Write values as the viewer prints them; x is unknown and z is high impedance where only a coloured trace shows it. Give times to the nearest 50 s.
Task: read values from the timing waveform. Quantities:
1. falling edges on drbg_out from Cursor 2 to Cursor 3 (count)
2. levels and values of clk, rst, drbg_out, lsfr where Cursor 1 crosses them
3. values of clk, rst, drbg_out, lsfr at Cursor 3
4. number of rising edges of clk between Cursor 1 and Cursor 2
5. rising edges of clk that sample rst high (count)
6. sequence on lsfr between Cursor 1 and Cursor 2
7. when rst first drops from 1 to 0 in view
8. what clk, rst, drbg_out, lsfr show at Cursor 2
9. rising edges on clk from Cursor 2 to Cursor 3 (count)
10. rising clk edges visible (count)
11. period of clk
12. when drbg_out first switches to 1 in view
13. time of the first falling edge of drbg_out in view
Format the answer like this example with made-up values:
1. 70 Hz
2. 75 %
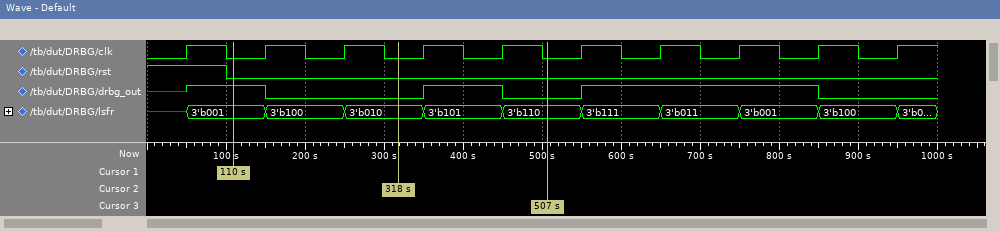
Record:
1. 1
2. clk=0, rst=0, drbg_out=1, lsfr=3'b001
3. clk=0, rst=0, drbg_out=0, lsfr=3'b110
4. 2
5. 1
6. 3'b001, 3'b100, 3'b010
7. 100 s
8. clk=0, rst=0, drbg_out=0, lsfr=3'b010
9. 2
10. 10
11. 100 s
12. 50 s
13. 150 s
